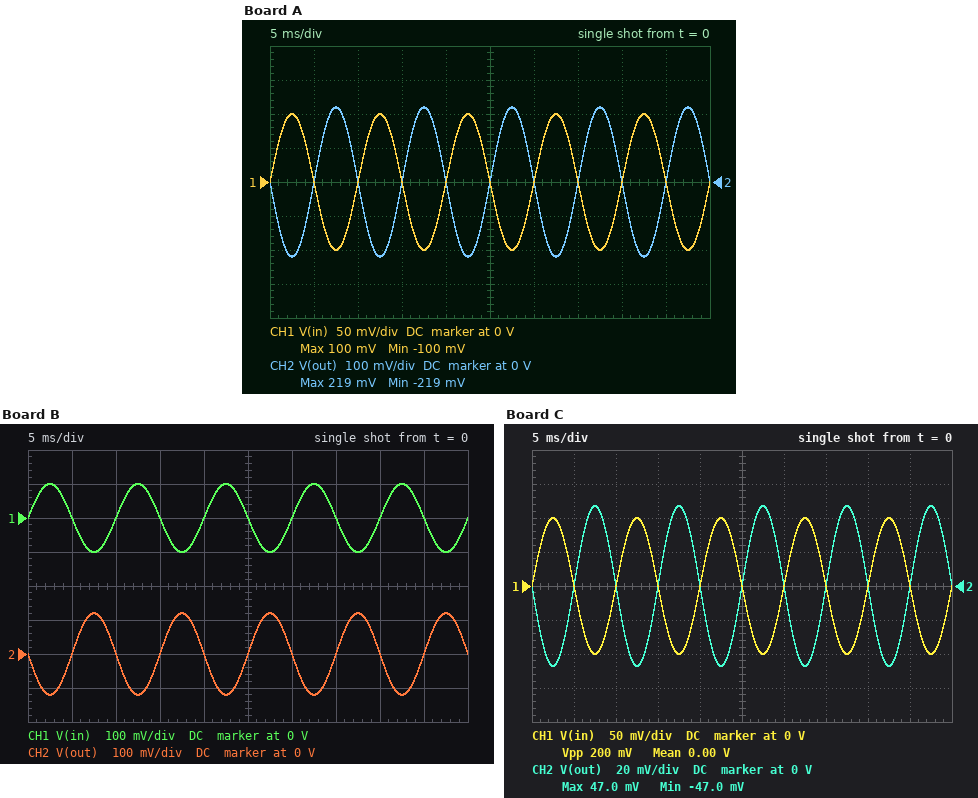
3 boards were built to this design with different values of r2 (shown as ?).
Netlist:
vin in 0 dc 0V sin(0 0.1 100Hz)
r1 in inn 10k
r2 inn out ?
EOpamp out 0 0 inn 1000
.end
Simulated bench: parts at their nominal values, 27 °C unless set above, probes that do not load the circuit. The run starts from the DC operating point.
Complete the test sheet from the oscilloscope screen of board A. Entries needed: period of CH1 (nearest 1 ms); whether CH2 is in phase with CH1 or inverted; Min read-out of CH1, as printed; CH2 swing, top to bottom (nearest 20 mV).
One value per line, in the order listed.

10 ms
inverted
-100 mV
440 mV
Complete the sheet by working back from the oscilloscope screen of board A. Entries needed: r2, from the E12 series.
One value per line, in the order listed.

22 kΩ
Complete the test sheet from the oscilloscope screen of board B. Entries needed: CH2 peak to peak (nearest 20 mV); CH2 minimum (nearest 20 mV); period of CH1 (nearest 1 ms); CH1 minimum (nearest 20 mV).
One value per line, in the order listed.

240 mV
-120 mV
10 ms
-100 mV
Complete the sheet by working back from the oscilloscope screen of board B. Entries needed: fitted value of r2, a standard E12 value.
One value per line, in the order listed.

12 kΩ
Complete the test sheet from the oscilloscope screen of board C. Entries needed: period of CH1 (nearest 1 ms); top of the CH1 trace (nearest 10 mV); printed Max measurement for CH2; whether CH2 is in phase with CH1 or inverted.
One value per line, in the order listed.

10 ms
100 mV
47.0 mV
inverted
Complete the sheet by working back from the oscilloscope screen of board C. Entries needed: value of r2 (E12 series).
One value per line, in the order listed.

4.7 kΩ
